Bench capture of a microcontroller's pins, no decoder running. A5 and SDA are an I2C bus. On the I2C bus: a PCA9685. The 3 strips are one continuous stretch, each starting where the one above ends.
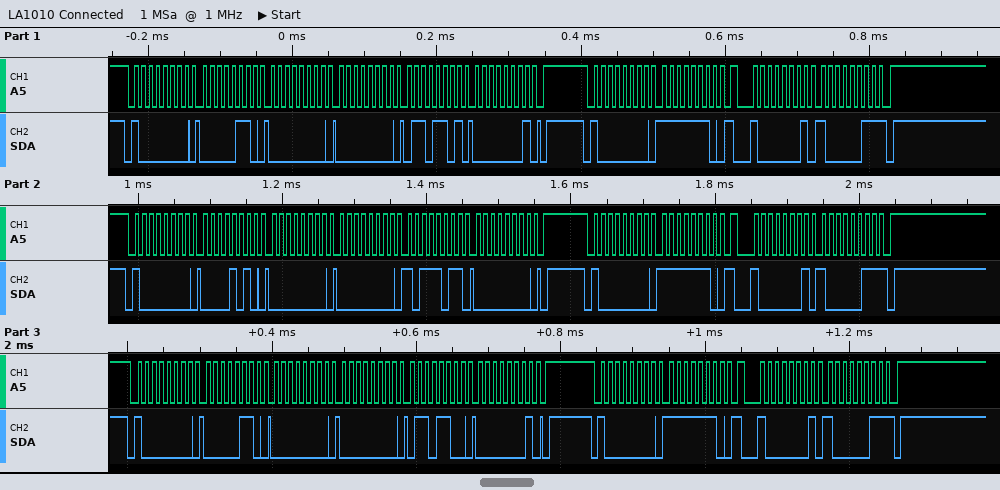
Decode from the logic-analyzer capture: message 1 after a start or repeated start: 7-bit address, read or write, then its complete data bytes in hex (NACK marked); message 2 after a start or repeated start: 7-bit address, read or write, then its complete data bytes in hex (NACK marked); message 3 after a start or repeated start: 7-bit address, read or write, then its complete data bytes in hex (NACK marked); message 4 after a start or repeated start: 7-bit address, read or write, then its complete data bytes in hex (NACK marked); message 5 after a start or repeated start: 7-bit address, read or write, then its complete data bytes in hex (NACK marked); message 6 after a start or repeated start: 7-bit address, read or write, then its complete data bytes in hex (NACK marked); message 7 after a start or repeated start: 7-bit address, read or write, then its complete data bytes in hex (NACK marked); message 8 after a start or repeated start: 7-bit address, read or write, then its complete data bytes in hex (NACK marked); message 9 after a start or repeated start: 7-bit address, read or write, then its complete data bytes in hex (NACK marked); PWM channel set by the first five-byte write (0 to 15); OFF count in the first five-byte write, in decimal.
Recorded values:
0x40 write: 06 00 00 6D 01
0x40 write: FE
0x40 read: 83 NACK
0x40 write: 0A 00 00 BB 00
0x40 write: FE
0x40 read: 83 NACK
0x40 write: 06 00 00 6C 01
0x40 write: FE
0x40 read: 83 NACK
0
365
